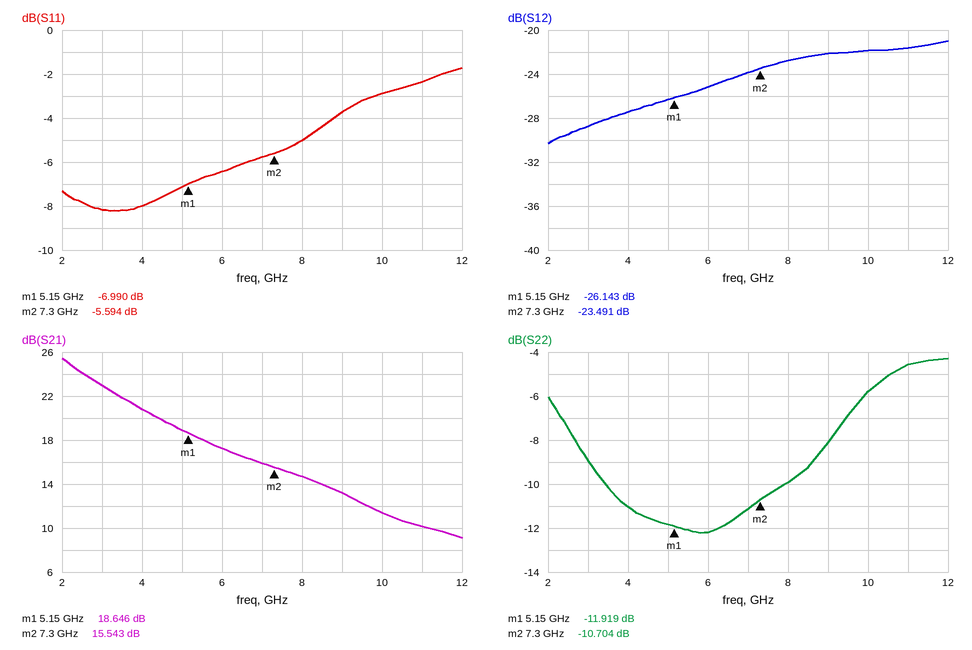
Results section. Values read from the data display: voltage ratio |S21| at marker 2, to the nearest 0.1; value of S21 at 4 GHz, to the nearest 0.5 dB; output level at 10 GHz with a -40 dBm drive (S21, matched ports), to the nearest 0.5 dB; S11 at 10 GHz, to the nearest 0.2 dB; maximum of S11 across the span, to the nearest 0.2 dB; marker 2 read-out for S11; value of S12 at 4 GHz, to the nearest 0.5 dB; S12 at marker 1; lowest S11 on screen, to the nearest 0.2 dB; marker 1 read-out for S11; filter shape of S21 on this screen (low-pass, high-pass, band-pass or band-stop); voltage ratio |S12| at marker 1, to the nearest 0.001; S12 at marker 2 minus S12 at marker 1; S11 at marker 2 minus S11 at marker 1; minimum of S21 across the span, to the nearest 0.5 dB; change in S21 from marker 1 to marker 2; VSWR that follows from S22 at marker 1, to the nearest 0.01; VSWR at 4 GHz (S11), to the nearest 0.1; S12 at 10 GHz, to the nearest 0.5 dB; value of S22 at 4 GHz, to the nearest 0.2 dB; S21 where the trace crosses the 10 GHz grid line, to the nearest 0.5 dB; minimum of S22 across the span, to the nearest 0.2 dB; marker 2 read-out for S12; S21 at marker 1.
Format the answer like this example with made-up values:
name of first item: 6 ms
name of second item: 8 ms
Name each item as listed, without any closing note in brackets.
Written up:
voltage ratio |S21| at marker 2, to the nearest 0.1: 6.0
value of S21 at 4 GHz, to the nearest 0.5 dB: 21.0 dB
output level at 10 GHz with a -40 dBm drive (S21, matched ports), to the nearest 0.5 dB: -28.5 dBm
S11 at 10 GHz, to the nearest 0.2 dB: -2.8 dB
maximum of S11 across the span, to the nearest 0.2 dB: -1.8 dB
marker 2 read-out for S11: -5.594 dB
value of S12 at 4 GHz, to the nearest 0.5 dB: -27.5 dB
S12 at marker 1: -26.143 dB
lowest S11 on screen, to the nearest 0.2 dB: -8.2 dB
marker 1 read-out for S11: -6.990 dB
filter shape of S21 on this screen: low-pass
voltage ratio |S12| at marker 1, to the nearest 0.001: 0.049
S12 at marker 2 minus S12 at marker 1: 2.652 dB
S11 at marker 2 minus S11 at marker 1: 1.396 dB
minimum of S21 across the span, to the nearest 0.5 dB: 9.0 dB
change in S21 from marker 1 to marker 2: -3.103 dB
VSWR that follows from S22 at marker 1, to the nearest 0.01: 1.68
VSWR at 4 GHz (S11), to the nearest 0.1: 2.3
S12 at 10 GHz, to the nearest 0.5 dB: -22.0 dB
value of S22 at 4 GHz, to the nearest 0.2 dB: -11.0 dB
S21 where the trace crosses the 10 GHz grid line, to the nearest 0.5 dB: 11.5 dB
minimum of S22 across the span, to the nearest 0.2 dB: -12.2 dB
marker 2 read-out for S12: -23.491 dB
S21 at marker 1: 18.646 dB
